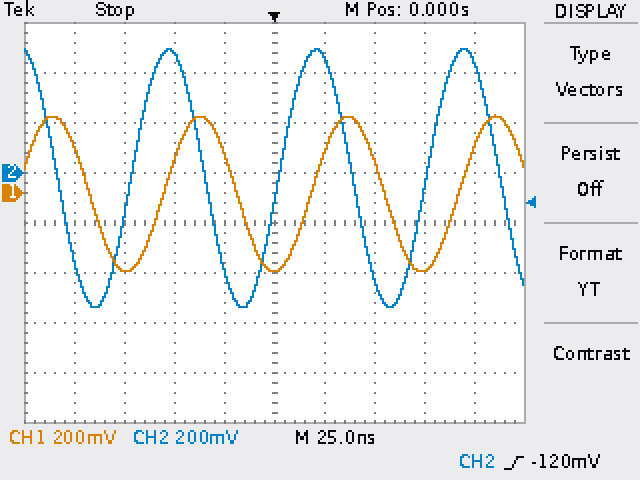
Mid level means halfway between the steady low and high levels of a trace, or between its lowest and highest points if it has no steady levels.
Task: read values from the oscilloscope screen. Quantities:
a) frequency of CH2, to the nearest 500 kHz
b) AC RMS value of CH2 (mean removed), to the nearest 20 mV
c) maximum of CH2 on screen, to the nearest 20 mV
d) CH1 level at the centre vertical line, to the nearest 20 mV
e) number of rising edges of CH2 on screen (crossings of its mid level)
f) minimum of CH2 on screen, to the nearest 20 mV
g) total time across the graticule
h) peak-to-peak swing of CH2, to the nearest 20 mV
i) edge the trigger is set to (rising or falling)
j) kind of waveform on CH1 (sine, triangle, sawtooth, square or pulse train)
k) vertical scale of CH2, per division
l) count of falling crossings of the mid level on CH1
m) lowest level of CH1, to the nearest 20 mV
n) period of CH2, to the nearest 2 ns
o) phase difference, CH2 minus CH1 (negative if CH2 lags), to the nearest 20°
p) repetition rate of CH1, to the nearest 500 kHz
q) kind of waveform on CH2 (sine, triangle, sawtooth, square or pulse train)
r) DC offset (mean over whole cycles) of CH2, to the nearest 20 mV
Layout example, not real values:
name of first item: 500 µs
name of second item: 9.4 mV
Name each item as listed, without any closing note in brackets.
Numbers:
frequency of CH2, to the nearest 500 kHz: 13.5 MHz
AC RMS value of CH2 (mean removed), to the nearest 20 mV: 360 mV
maximum of CH2 on screen, to the nearest 20 mV: 500 mV
CH1 level at the centre vertical line, to the nearest 20 mV: -320 mV
number of rising edges of CH2 on screen: 3
minimum of CH2 on screen, to the nearest 20 mV: -540 mV
total time across the graticule: 250 ns
peak-to-peak swing of CH2, to the nearest 20 mV: 1.04 V
edge the trigger is set to: rising
kind of waveform on CH1: sine
vertical scale of CH2, per division: 200 mV
count of falling crossings of the mid level on CH1: 3
lowest level of CH1, to the nearest 20 mV: -320 mV
period of CH2, to the nearest 2 ns: 74 ns
phase difference, CH2 minus CH1 (negative if CH2 lags), to the nearest 20°: +80°
repetition rate of CH1, to the nearest 500 kHz: 13.5 MHz
kind of waveform on CH2: sine
DC offset (mean over whole cycles) of CH2, to the nearest 20 mV: -20 mV
